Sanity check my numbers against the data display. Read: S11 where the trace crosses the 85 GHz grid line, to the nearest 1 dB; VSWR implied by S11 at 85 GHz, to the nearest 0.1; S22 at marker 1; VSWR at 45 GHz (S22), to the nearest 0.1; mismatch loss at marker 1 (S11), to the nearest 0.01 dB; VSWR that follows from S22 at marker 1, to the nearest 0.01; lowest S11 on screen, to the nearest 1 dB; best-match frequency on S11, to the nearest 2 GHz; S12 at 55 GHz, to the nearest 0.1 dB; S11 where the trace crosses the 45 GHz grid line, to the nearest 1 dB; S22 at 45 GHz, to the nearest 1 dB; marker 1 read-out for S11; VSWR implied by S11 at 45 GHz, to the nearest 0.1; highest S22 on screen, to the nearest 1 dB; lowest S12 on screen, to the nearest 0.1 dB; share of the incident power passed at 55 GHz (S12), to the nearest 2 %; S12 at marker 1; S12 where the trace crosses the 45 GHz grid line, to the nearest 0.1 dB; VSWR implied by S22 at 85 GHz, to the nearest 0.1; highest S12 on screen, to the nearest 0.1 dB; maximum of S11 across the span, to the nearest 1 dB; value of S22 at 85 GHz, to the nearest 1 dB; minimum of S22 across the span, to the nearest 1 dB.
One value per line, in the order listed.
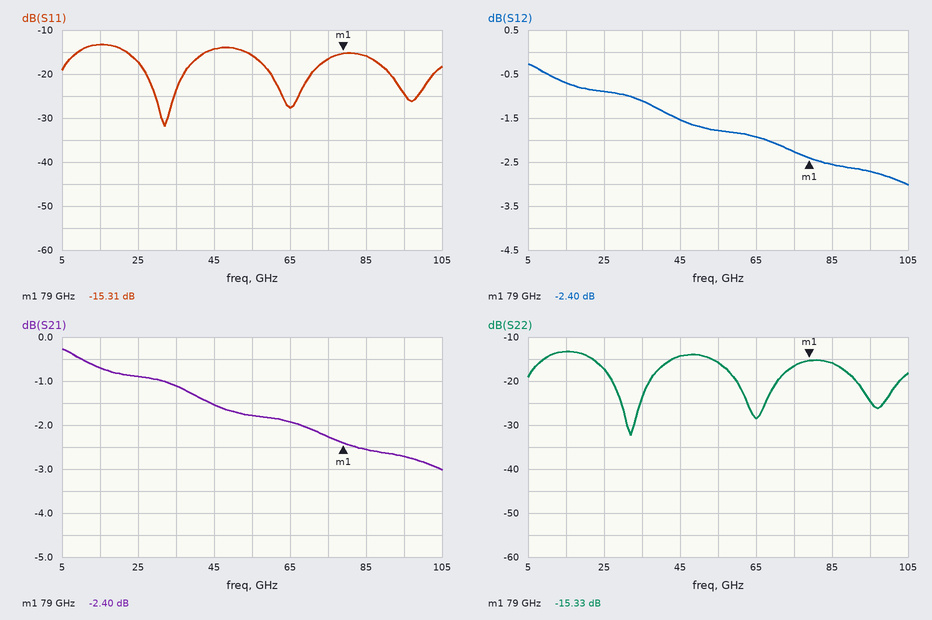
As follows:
-16 dB
1.4
-15.33 dB
1.5
0.13 dB
1.41
-32 dB
32 GHz
-1.8 dB
-14 dB
-14 dB
-15.31 dB
1.5
-13 dB
-3.0 dB
66 %
-2.40 dB
-1.5 dB
1.4
-0.3 dB
-13 dB
-16 dB
-32 dB
